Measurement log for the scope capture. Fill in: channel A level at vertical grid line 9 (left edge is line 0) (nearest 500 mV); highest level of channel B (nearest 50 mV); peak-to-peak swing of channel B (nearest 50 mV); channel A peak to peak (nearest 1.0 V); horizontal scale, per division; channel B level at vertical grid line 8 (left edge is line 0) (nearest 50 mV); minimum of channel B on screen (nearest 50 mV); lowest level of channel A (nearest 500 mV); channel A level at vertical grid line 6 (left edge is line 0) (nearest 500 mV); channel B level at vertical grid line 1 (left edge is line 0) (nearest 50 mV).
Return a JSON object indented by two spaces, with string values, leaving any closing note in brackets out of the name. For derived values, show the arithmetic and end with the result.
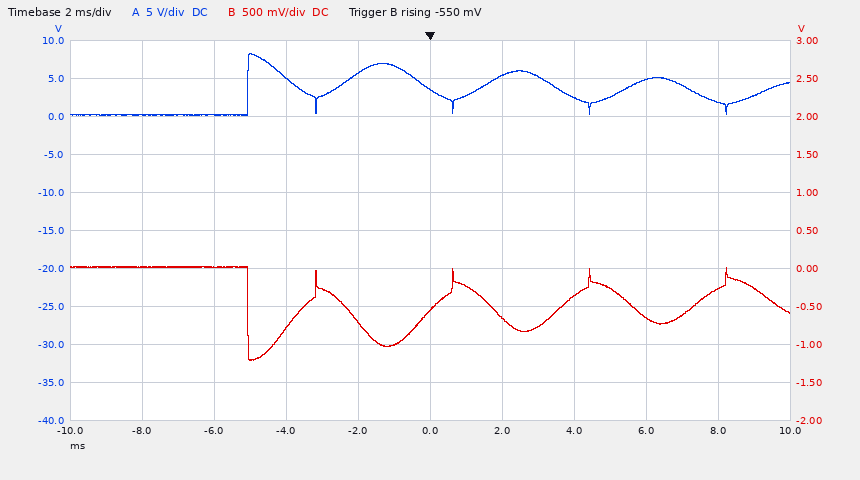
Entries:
{
  "channel A level at vertical grid line 9 (left edge is line 0)": "2.0 V",
  "highest level of channel B": "50 mV",
  "peak-to-peak swing of channel B": "50 mV − (-1.20 V) = 1.25 V",
  "channel A peak to peak": "8.0 V",
  "horizontal scale, per division": "2 ms",
  "channel B level at vertical grid line 8 (left edge is line 0)": "-650 mV",
  "minimum of channel B on screen": "-1.20 V",
  "lowest level of channel A": "0.0 V",
  "channel A level at vertical grid line 6 (left edge is line 0)": "5.5 V",
  "channel B level at vertical grid line 1 (left edge is line 0)": "0 mV"
}
